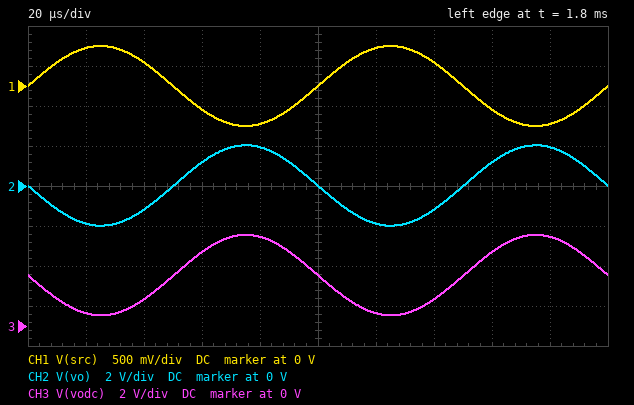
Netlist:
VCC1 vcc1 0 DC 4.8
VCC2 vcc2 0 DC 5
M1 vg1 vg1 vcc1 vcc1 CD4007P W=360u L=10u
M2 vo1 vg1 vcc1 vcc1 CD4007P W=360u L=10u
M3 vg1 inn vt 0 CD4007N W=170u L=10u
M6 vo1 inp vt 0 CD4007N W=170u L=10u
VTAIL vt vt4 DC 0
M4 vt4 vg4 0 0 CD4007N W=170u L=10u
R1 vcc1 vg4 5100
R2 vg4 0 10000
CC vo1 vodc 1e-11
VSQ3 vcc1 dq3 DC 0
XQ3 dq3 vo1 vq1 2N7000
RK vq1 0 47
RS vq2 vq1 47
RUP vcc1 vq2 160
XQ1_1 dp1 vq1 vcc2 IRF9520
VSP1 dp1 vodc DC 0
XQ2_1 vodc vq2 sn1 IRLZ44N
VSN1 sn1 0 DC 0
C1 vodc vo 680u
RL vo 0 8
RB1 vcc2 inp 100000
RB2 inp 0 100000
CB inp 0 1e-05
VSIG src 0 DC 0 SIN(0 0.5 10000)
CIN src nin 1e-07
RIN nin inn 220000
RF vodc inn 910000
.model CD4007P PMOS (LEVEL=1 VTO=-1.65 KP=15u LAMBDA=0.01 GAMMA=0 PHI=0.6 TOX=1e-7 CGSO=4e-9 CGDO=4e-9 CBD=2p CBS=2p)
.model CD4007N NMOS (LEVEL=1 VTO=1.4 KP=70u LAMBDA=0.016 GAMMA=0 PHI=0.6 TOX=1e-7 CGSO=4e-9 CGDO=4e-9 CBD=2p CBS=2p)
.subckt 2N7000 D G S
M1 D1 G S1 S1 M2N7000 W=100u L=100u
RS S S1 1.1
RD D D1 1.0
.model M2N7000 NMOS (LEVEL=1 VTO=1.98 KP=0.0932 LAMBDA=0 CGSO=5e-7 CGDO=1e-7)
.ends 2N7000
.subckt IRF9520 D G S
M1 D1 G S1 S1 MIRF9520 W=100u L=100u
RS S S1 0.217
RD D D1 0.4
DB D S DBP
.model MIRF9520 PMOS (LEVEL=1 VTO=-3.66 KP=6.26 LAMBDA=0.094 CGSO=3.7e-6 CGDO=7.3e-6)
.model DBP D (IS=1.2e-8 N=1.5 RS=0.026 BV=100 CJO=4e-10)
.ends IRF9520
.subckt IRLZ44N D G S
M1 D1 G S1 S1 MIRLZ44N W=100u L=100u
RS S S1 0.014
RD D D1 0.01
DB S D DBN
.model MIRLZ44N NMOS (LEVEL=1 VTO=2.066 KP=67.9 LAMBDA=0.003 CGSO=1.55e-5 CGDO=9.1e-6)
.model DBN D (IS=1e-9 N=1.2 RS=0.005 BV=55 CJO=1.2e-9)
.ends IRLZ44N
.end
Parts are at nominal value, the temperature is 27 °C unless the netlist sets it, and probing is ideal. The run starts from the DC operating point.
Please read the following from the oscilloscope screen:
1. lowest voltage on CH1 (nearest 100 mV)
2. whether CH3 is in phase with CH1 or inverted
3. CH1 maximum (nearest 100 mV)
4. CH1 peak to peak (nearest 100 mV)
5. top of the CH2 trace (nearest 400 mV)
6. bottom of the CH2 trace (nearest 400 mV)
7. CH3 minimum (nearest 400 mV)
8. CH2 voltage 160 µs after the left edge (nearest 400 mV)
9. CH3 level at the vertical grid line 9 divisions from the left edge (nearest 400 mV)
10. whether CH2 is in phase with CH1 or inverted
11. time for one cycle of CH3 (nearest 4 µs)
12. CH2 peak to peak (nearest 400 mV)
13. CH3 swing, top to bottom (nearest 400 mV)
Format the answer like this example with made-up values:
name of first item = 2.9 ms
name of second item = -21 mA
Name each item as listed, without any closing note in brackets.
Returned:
lowest voltage on CH1 = -500 mV
whether CH3 is in phase with CH1 or inverted = inverted
CH1 maximum = 500 mV
CH1 peak to peak = 1.0 V
top of the CH2 trace = 2.0 V
bottom of the CH2 trace = -2.0 V
CH3 minimum = 400 mV
CH2 voltage 160 µs after the left edge = 1.2 V
CH3 level at the vertical grid line 9 divisions from the left edge = 4.4 V
whether CH2 is in phase with CH1 or inverted = inverted
time for one cycle of CH3 = 100 µs
CH2 peak to peak = 4.0 V
CH3 swing, top to bottom = 4.0 V
